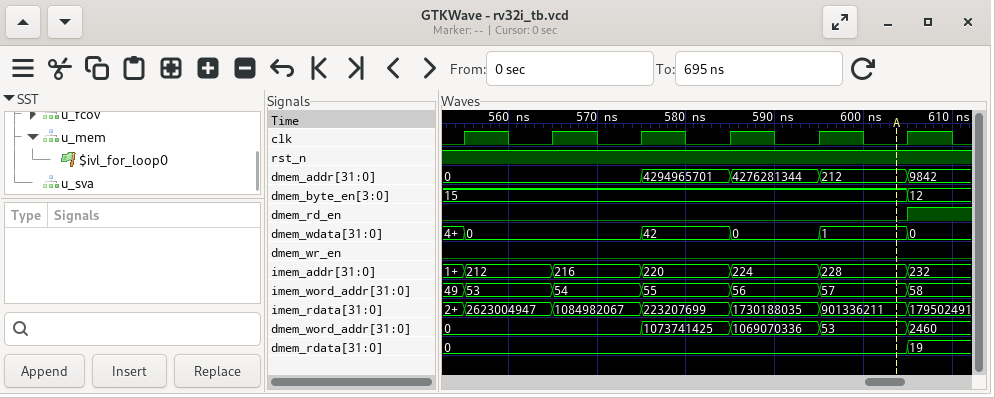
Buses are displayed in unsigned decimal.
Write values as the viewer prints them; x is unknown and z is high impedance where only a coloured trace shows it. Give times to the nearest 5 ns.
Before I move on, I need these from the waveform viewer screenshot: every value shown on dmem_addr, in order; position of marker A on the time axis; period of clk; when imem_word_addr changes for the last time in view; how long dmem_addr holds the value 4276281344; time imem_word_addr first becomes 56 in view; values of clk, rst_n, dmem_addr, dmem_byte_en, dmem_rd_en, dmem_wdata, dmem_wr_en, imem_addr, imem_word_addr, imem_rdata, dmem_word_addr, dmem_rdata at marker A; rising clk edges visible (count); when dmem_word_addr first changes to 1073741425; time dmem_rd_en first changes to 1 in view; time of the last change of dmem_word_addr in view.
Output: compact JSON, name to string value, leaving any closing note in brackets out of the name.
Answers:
{"every value shown on dmem_addr, in order": "0, 4294965701, 4276281344, 212, 9842", "position of marker A on the time axis": "605 ns", "period of clk": "10 ns", "when imem_word_addr changes for the last time in view": "605 ns", "how long dmem_addr holds the value 4276281344": "10 ns", "time imem_word_addr first becomes 56 in view": "585 ns", "values of clk, rst_n, dmem_addr, dmem_byte_en, dmem_rd_en, dmem_wdata, dmem_wr_en, imem_addr, imem_word_addr, imem_rdata, dmem_word_addr, dmem_rdata at marker A": "clk=0, rst_n=1, dmem_addr=212, dmem_byte_en=15, dmem_rd_en=0, dmem_wdata=1, dmem_wr_en=0, imem_addr=228, imem_word_addr=57, imem_rdata=901336211, dmem_word_addr=53, dmem_rdata=0", "rising clk edges visible": "6", "when dmem_word_addr first changes to 1073741425": "575 ns", "time dmem_rd_en first changes to 1 in view": "605 ns", "time of the last change of dmem_word_addr in view": "605 ns"}
